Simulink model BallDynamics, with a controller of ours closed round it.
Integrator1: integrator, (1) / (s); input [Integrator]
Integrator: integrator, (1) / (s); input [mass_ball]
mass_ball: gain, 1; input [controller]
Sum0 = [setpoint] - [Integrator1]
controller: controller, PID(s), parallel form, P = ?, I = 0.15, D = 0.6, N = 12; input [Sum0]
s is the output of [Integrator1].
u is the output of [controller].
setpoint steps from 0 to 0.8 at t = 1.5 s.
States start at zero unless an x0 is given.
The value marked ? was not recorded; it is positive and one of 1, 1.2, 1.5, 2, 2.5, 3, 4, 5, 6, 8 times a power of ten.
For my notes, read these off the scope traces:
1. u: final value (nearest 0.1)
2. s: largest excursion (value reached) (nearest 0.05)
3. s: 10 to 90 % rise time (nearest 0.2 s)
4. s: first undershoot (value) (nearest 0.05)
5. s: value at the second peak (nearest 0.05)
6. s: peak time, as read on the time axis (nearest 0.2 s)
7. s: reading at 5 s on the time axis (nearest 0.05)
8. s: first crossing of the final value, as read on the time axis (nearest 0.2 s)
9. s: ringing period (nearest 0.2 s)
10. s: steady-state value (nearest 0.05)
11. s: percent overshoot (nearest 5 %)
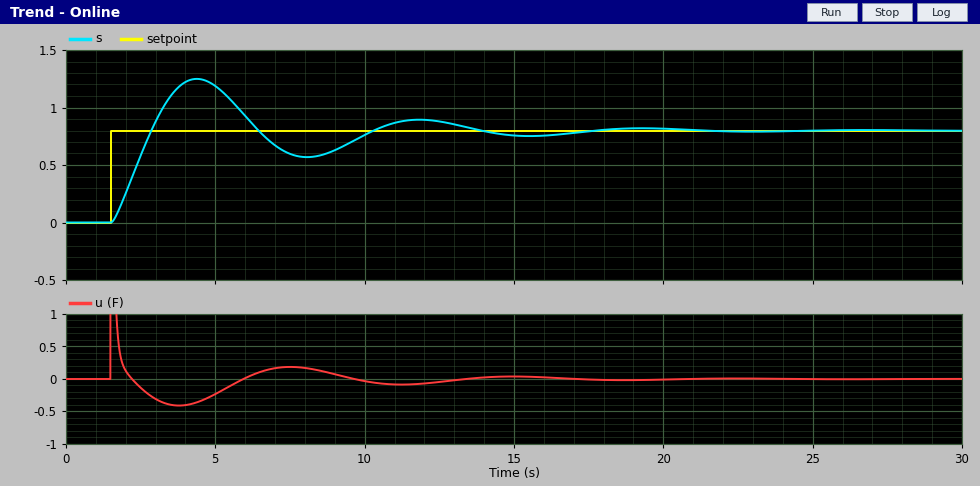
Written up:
0.0
1.25
1.0 s
0.55
0.90
4.4 s
1.20
2.8 s
7.4 s
0.80
55 %
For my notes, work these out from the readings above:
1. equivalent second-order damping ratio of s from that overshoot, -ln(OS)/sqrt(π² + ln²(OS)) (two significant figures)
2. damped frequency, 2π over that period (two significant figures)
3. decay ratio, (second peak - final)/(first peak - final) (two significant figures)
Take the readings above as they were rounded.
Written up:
0.19
0.85 rad/s
0.22
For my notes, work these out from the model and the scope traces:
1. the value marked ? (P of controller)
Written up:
0.8
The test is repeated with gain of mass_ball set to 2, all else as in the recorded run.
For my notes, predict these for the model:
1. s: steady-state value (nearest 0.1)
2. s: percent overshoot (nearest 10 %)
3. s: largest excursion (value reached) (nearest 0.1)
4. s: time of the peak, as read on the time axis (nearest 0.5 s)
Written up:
0.8
40 %
1.1
3.5 s
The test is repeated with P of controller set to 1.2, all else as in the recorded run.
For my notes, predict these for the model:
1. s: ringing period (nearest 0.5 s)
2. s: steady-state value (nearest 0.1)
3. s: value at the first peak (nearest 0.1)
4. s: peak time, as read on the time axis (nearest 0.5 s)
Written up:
6.0 s
0.8
1.3
4.0 s
